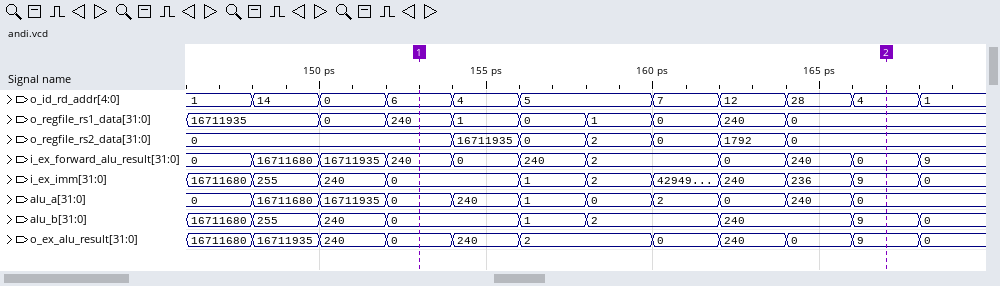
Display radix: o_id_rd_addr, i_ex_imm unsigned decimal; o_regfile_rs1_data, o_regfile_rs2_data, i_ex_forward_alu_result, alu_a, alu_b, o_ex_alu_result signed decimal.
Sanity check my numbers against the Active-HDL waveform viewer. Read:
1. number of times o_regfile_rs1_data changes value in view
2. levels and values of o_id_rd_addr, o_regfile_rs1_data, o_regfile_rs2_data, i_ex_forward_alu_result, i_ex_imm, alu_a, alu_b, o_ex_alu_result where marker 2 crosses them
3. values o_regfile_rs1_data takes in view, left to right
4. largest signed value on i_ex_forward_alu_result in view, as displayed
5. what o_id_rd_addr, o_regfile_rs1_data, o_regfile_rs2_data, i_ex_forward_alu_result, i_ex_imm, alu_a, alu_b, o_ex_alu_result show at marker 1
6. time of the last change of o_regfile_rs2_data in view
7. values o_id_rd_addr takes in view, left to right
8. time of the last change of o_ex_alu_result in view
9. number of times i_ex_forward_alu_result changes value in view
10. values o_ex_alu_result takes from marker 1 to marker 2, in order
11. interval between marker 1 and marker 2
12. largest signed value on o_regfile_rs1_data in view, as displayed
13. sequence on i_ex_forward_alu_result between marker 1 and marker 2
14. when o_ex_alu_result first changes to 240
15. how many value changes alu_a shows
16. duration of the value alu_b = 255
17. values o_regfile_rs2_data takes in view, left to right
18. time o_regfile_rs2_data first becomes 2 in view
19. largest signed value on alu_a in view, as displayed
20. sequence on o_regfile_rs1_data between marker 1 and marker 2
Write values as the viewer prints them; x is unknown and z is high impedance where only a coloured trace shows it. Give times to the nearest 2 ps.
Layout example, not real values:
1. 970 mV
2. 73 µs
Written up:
1. 8
2. o_id_rd_addr=4, o_regfile_rs1_data=0, o_regfile_rs2_data=0, i_ex_forward_alu_result=0, i_ex_imm=9, alu_a=0, alu_b=9, o_ex_alu_result=9
3. 16711935, 0, 240, 1, 0, 1, 0, 240, 0
4. 16711935
5. o_id_rd_addr=6, o_regfile_rs1_data=240, o_regfile_rs2_data=0, i_ex_forward_alu_result=240, i_ex_imm=0, alu_a=0, alu_b=0, o_ex_alu_result=0
6. 164 ps
7. 1, 14, 0, 6, 4, 5, 7, 12, 28, 4, 1
8. 168 ps
9. 10
10. 0, 240, 2, 0, 240, 0, 9
11. 14 ps
12. 16711935
13. 240, 0, 240, 2, 0, 240, 0
14. 150 ps
15. 10
16. 2 ps
17. 0, 16711935, 0, 2, 0, 1792, 0
18. 158 ps
19. 16711935
20. 240, 1, 0, 1, 0, 240, 0
